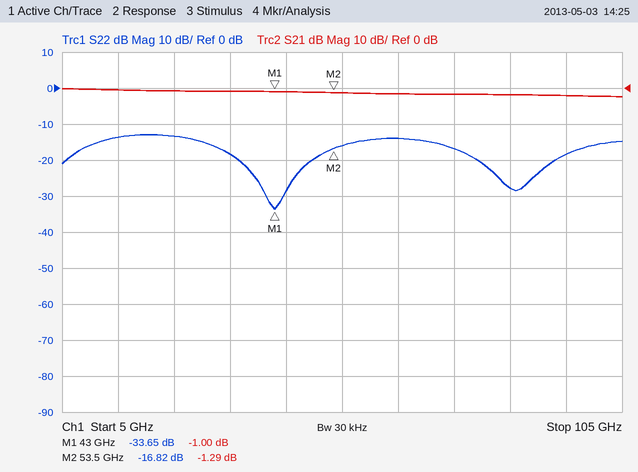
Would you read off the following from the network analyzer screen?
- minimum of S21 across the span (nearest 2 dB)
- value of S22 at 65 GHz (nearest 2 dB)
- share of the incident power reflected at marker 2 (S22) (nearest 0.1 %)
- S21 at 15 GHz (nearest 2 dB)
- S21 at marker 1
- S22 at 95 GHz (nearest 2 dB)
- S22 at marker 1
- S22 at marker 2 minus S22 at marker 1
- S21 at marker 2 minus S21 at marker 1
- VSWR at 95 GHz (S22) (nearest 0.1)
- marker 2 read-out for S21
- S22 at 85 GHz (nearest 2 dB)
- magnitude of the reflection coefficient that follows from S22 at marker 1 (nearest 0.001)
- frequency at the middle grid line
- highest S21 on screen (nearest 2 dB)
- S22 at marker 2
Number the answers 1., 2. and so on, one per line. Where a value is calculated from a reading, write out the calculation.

1. -2 dB
2. -14 dB
3. 10^(-16.82/10) ≈ 2.1 %
4. 0 dB
5. -1.00 dB
6. -18 dB
7. -33.65 dB
8. -16.82 − (-33.65) = 16.83 dB
9. -1.29 − (-1) = -0.29 dB
10. |Γ| = 10^(-18/20) = 0.1259; VSWR = (1 + 0.1259)/(1 − 0.1259) ≈ 1.3
11. -1.29 dB
12. -28 dB
13. 10^(-33.65/20) ≈ 0.021
14. 55 GHz
15. 0 dB
16. -16.82 dB
